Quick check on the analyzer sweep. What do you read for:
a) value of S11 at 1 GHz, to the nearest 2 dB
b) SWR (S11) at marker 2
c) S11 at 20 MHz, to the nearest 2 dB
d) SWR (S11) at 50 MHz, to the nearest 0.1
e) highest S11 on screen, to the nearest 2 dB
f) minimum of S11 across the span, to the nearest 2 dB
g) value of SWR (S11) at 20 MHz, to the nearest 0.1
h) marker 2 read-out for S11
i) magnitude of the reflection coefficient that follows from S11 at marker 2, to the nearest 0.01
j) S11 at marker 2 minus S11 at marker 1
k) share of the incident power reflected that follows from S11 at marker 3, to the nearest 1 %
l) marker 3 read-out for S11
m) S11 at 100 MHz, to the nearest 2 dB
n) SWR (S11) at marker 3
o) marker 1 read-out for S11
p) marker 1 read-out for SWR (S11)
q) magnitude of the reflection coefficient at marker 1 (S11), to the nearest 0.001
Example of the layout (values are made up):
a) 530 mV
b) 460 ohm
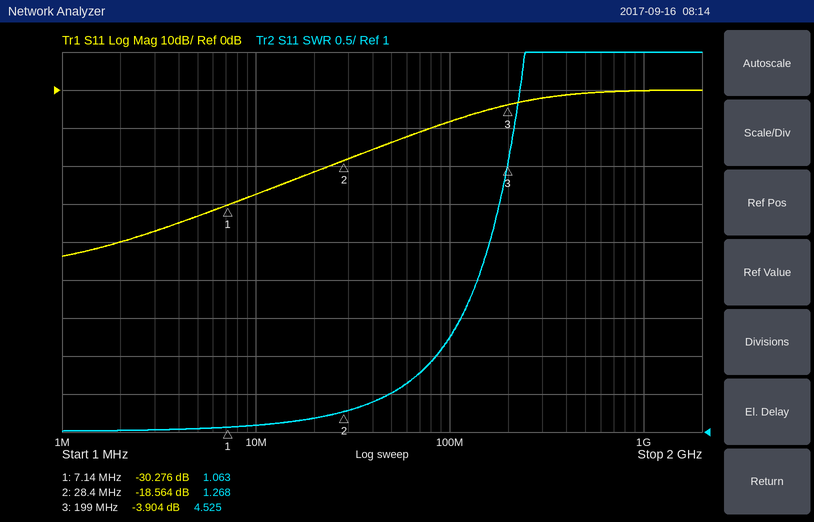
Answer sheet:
a) 0 dB
b) 1.268
c) -22 dB
d) 1.5
e) 0 dB
f) -44 dB
g) 1.2
h) -18.564 dB
i) 0.12
j) 11.712 dB
k) 41 %
l) -3.904 dB
m) -8 dB
n) 4.525
o) -30.276 dB
p) 1.063
q) 0.031
